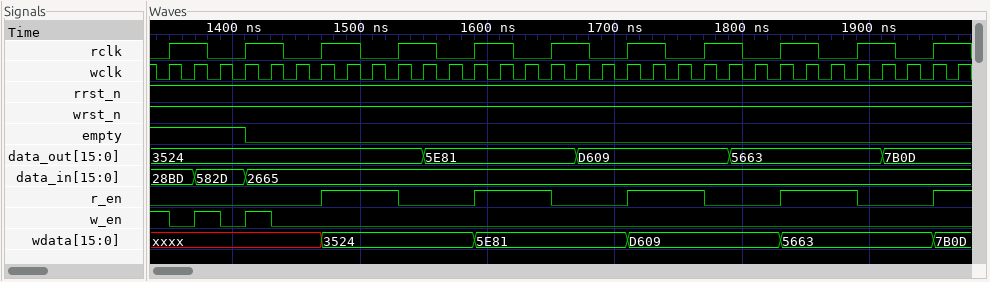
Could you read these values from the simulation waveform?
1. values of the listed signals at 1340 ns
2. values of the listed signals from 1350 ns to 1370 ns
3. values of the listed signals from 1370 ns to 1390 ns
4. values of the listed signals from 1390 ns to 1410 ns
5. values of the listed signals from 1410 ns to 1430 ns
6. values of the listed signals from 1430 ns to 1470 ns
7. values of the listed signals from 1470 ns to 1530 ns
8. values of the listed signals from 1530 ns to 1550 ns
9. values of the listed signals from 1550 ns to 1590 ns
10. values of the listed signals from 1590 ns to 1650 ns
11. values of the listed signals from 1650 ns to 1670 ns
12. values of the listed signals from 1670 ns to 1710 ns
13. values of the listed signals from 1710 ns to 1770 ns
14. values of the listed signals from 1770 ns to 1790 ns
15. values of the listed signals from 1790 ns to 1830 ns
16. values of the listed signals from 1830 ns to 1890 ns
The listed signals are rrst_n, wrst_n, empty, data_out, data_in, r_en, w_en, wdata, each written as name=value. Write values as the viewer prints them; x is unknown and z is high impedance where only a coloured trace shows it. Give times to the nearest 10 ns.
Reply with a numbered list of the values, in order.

1. rrst_n=1, wrst_n=1, empty=1, data_out=3524, data_in=28BD, r_en=0, w_en=1, wdata=xxxx
2. rrst_n=1, wrst_n=1, empty=1, data_out=3524, data_in=28BD, r_en=0, w_en=0, wdata=xxxx
3. rrst_n=1, wrst_n=1, empty=1, data_out=3524, data_in=582D, r_en=0, w_en=1, wdata=xxxx
4. rrst_n=1, wrst_n=1, empty=1, data_out=3524, data_in=582D, r_en=0, w_en=0, wdata=xxxx
5. rrst_n=1, wrst_n=1, empty=0, data_out=3524, data_in=2665, r_en=0, w_en=1, wdata=xxxx
6. rrst_n=1, wrst_n=1, empty=0, data_out=3524, data_in=2665, r_en=0, w_en=0, wdata=xxxx
7. rrst_n=1, wrst_n=1, empty=0, data_out=3524, data_in=2665, r_en=1, w_en=0, wdata=3524
8. rrst_n=1, wrst_n=1, empty=0, data_out=3524, data_in=2665, r_en=0, w_en=0, wdata=3524
9. rrst_n=1, wrst_n=1, empty=0, data_out=5E81, data_in=2665, r_en=0, w_en=0, wdata=3524
10. rrst_n=1, wrst_n=1, empty=0, data_out=5E81, data_in=2665, r_en=1, w_en=0, wdata=5E81
11. rrst_n=1, wrst_n=1, empty=0, data_out=5E81, data_in=2665, r_en=0, w_en=0, wdata=5E81
12. rrst_n=1, wrst_n=1, empty=0, data_out=D609, data_in=2665, r_en=0, w_en=0, wdata=5E81
13. rrst_n=1, wrst_n=1, empty=0, data_out=D609, data_in=2665, r_en=1, w_en=0, wdata=D609
14. rrst_n=1, wrst_n=1, empty=0, data_out=D609, data_in=2665, r_en=0, w_en=0, wdata=D609
15. rrst_n=1, wrst_n=1, empty=0, data_out=5663, data_in=2665, r_en=0, w_en=0, wdata=D609
16. rrst_n=1, wrst_n=1, empty=0, data_out=5663, data_in=2665, r_en=1, w_en=0, wdata=5663
